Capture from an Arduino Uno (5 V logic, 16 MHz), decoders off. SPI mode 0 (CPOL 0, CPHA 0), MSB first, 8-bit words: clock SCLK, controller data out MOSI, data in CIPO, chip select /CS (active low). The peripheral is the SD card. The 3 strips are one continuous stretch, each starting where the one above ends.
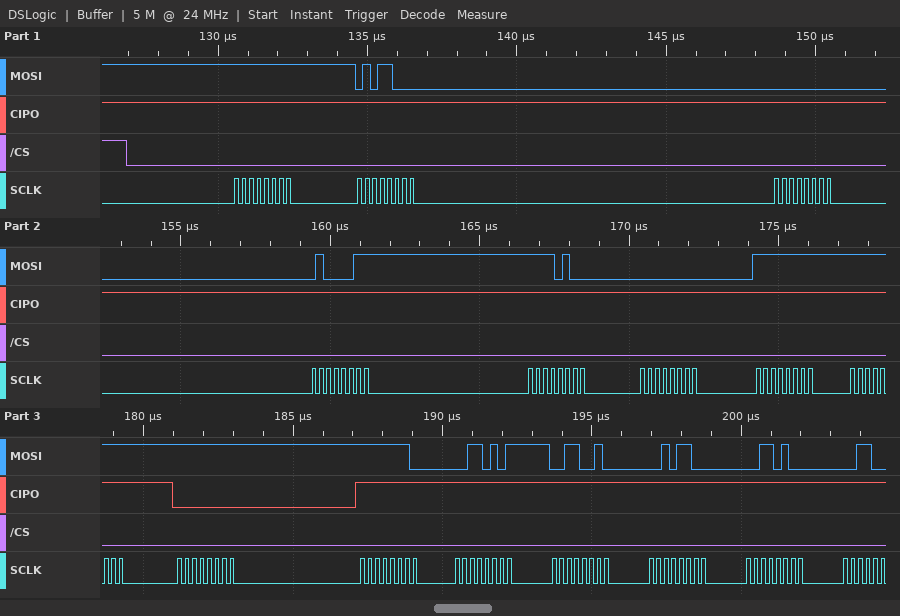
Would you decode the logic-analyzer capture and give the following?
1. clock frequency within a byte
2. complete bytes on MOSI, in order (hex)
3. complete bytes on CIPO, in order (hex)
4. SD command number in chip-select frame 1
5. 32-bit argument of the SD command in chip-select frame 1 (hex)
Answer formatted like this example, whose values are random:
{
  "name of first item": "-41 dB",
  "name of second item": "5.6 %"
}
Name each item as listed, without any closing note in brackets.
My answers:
{
  "clock frequency within a byte": "4 MHz",
  "complete bytes on MOSI, in order": "0xFF 0x58 0x00 0x43 0xF4 0x00 0xFF 0xFF 0xFF 0xFE 0x35 0x32 0x2C 0x34",
  "complete bytes on CIPO, in order": "0xFF 0xFF 0xFF 0xFF 0xFF 0xFF 0xFF 0xFF 0x00 0xFF 0xFF 0xFF 0xFF 0xFF",
  "SD command number in chip-select frame 1": "CMD24",
  "32-bit argument of the SD command in chip-select frame 1": "0x0043F400"
}
